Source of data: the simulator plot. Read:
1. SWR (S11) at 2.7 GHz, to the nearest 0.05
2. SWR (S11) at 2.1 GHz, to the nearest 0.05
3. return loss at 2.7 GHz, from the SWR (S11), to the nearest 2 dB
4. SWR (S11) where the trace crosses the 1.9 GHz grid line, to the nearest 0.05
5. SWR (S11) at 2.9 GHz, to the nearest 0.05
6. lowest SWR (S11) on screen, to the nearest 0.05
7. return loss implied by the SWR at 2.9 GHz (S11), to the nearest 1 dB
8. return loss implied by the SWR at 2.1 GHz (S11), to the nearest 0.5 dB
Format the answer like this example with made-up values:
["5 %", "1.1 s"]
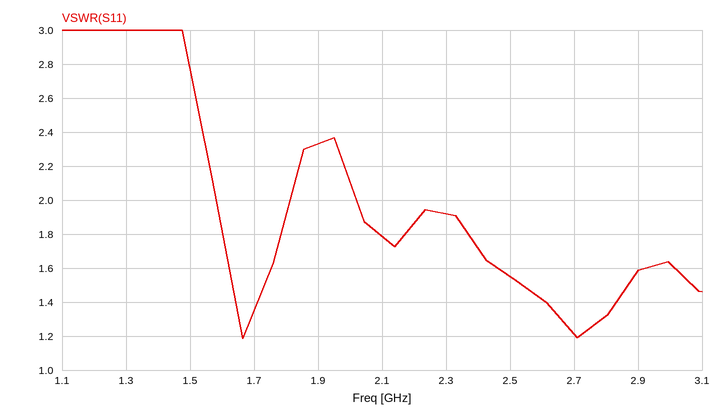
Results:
["1.20", "1.80", "20 dB", "2.35", "1.60", "1.20", "13 dB", "11.0 dB"]
